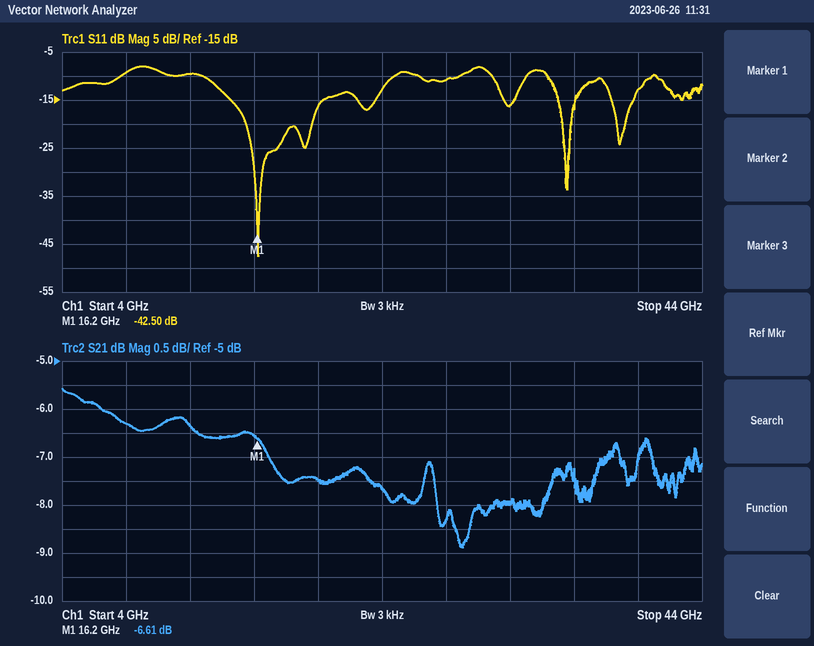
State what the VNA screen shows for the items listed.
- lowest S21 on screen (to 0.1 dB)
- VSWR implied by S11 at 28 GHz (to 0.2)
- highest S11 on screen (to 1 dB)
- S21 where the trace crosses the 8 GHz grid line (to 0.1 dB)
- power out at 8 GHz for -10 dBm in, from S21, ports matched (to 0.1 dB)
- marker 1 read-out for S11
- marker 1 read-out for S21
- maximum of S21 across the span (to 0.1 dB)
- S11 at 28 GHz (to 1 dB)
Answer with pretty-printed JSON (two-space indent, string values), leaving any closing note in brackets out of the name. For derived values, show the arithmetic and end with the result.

{
  "lowest S21 on screen": "-8.9 dB",
  "VSWR implied by S11 at 28 GHz": "|Γ| = 10^(-11/20) = 0.2818; VSWR = (1 + 0.2818)/(1 − 0.2818) ≈ 1.8",
  "highest S11 on screen": "-8 dB",
  "S21 where the trace crosses the 8 GHz grid line": "-6.3 dB",
  "power out at 8 GHz for -10 dBm in, from S21, ports matched": "-10 dBm + (-6.3 dB) = -16.3 dBm",
  "marker 1 read-out for S11": "-42.50 dB",
  "marker 1 read-out for S21": "-6.61 dB",
  "maximum of S21 across the span": "-5.6 dB",
  "S11 at 28 GHz": "-11 dB"
}
